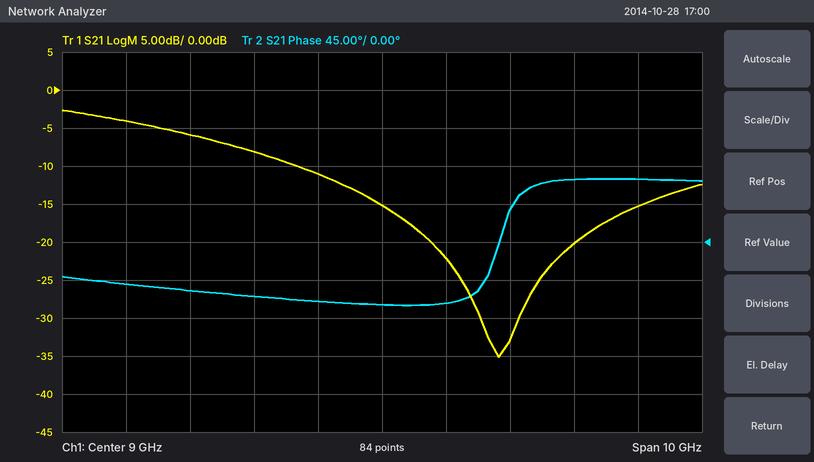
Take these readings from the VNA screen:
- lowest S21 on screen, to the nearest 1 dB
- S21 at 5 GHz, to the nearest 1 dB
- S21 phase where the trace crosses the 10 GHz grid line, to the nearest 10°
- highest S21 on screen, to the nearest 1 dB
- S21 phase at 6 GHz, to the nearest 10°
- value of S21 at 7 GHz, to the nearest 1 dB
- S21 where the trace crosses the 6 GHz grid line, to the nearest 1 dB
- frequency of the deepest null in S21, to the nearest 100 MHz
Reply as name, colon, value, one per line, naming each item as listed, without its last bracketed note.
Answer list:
lowest S21 on screen, to the nearest 1 dB: -35 dB
S21 at 5 GHz, to the nearest 1 dB: -4 dB
S21 phase where the trace crosses the 10 GHz grid line, to the nearest 10°: -70°
highest S21 on screen, to the nearest 1 dB: -3 dB
S21 phase at 6 GHz, to the nearest 10°: -60°
value of S21 at 7 GHz, to the nearest 1 dB: -8 dB
S21 where the trace crosses the 6 GHz grid line, to the nearest 1 dB: -6 dB
frequency of the deepest null in S21, to the nearest 100 MHz: 10.8 GHz
